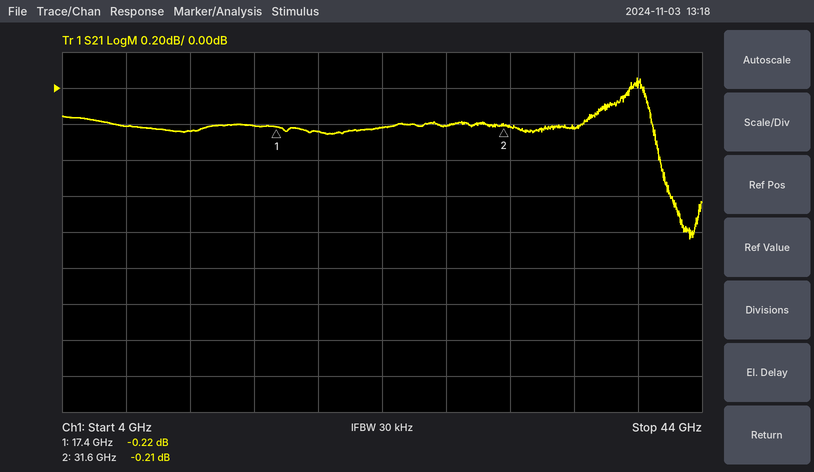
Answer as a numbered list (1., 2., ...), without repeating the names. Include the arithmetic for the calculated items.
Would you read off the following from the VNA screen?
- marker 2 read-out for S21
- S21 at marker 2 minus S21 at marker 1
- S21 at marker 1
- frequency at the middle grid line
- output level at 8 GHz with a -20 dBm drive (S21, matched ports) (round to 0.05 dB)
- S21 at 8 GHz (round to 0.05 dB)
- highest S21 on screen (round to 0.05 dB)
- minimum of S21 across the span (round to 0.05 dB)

1. -0.21 dB
2. -0.21 − (-0.22) = 0.01 dB
3. -0.22 dB
4. 24 GHz
5. -20 dBm + (-0.20 dB) = -20.20 dBm
6. -0.20 dB
7. 0.05 dB
8. -0.85 dB
